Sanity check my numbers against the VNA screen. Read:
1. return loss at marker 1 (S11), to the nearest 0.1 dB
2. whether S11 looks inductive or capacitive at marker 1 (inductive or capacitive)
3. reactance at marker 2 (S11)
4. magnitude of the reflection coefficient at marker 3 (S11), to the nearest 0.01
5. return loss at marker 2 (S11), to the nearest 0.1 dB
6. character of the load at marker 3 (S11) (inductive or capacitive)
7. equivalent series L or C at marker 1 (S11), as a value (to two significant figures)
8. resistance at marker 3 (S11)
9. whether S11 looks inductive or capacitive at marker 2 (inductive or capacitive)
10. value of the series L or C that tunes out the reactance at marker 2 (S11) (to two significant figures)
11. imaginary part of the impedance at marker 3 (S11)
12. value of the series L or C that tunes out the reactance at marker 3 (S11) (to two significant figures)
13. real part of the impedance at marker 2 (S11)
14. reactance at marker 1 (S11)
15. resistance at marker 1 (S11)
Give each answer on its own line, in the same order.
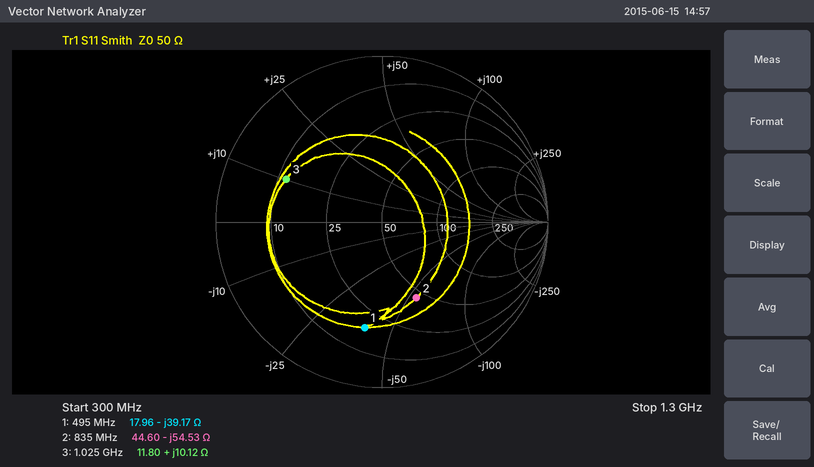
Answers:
3.8 dB
capacitive
-54.53 Ω
0.63
6.0 dB
inductive
8.2 pF
11.80 Ω
capacitive
10 nH
+10.12 Ω
15 pF
44.60 Ω
-39.17 Ω
17.96 Ω
